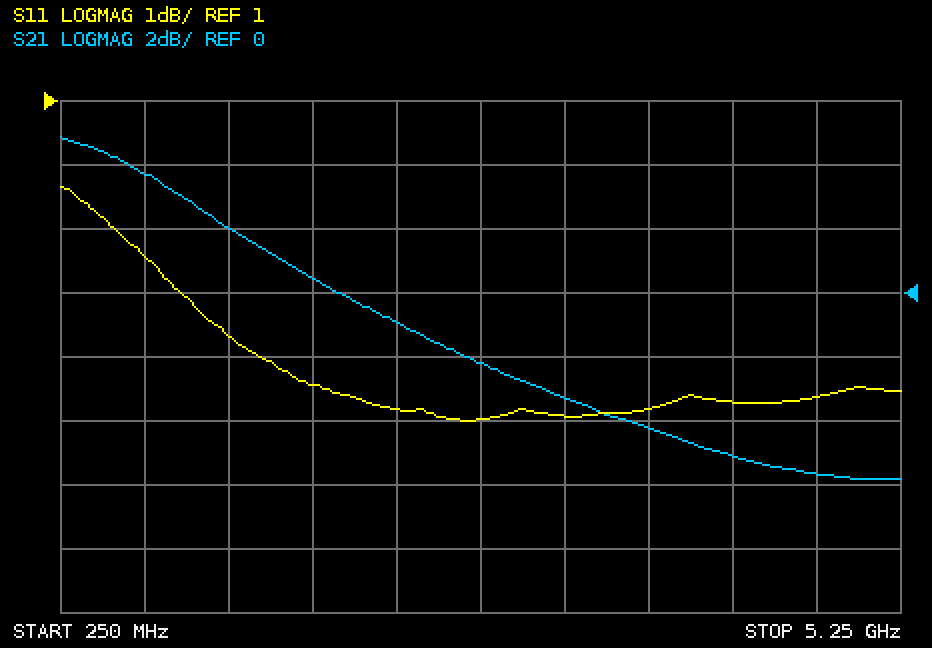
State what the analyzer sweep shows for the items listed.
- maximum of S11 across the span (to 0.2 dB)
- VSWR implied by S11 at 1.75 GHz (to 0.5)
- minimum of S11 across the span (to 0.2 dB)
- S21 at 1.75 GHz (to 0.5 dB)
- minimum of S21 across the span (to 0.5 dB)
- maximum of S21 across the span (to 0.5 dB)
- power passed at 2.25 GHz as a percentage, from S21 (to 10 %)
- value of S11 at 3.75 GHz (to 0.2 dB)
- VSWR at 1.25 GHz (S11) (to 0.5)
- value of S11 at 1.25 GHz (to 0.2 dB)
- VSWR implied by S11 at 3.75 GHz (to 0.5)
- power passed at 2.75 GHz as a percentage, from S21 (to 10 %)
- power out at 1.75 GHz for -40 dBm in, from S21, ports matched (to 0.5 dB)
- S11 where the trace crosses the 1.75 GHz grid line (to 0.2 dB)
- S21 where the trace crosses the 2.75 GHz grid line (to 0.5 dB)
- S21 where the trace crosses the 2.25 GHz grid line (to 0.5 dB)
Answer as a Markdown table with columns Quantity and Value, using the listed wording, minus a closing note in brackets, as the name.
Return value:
| Quantity | Value |
|---|---|
| maximum of S11 across the span | -0.4 dB |
| VSWR implied by S11 at 1.75 GHz | 5.0 |
| minimum of S11 across the span | -4.0 dB |
| S21 at 1.75 GHz | 0.5 dB |
| minimum of S21 across the span | -6.0 dB |
| maximum of S21 across the span | 5.0 dB |
| power passed at 2.25 GHz as a percentage, from S21 | 80 % |
| value of S11 at 3.75 GHz | -3.8 dB |
| VSWR at 1.25 GHz (S11) | 6.5 |
| value of S11 at 1.25 GHz | -2.6 dB |
| VSWR implied by S11 at 3.75 GHz | 4.5 |
| power passed at 2.75 GHz as a percentage, from S21 | 60 % |
| power out at 1.75 GHz for -40 dBm in, from S21, ports matched | -39.5 dBm |
| S11 where the trace crosses the 1.75 GHz grid line | -3.4 dB |
| S21 where the trace crosses the 2.75 GHz grid line | -2.0 dB |
| S21 where the trace crosses the 2.25 GHz grid line | -1.0 dB |
